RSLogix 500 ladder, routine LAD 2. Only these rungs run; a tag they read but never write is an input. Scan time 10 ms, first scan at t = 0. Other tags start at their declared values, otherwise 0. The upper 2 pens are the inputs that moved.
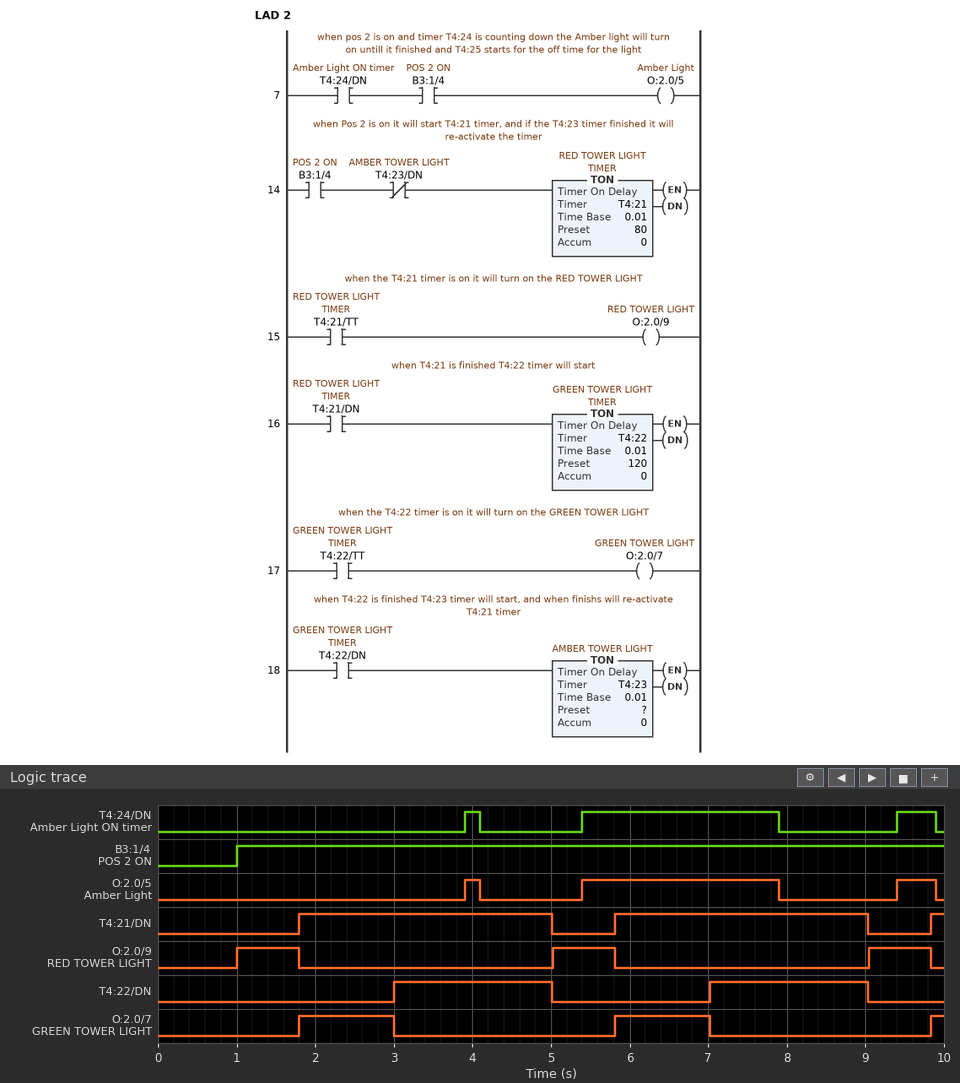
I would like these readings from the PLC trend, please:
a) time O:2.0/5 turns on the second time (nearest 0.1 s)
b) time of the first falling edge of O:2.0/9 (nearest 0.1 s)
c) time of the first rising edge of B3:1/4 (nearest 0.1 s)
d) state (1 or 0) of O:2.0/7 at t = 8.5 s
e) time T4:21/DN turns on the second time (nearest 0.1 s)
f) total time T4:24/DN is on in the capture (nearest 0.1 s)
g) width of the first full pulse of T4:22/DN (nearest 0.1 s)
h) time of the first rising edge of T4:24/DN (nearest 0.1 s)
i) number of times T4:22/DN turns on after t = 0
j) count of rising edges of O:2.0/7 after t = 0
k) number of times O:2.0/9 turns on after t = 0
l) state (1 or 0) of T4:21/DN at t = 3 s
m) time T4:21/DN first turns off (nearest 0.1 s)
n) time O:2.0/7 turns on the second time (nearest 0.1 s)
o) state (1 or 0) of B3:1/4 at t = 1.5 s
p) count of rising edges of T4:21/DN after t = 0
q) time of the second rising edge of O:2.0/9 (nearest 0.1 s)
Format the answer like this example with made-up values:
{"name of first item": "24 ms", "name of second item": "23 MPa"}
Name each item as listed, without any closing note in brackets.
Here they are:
{"time O:2.0/5 turns on the second time": "5.4 s", "time of the first falling edge of O:2.0/9": "1.8 s", "time of the first rising edge of B3:1/4": "1.0 s", "state (1 or 0) of O:2.0/7 at t = 8.5 s": "0", "time T4:21/DN turns on the second time": "5.8 s", "total time T4:24/DN is on in the capture": "3.2 s", "width of the first full pulse of T4:22/DN": "2.0 s", "time of the first rising edge of T4:24/DN": "3.9 s", "number of times T4:22/DN turns on after t = 0": "2", "count of rising edges of O:2.0/7 after t = 0": "3", "number of times O:2.0/9 turns on after t = 0": "3", "state (1 or 0) of T4:21/DN at t = 3 s": "1", "time T4:21/DN first turns off": "5.0 s", "time O:2.0/7 turns on the second time": "5.8 s", "state (1 or 0) of B3:1/4 at t = 1.5 s": "1", "count of rising edges of T4:21/DN after t = 0": "3", "time of the second rising edge of O:2.0/9": "5.0 s"}
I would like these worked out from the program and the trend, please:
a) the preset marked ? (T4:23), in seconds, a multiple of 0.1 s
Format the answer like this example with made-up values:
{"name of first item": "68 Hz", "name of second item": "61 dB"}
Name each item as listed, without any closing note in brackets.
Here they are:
{"the preset marked ? (T4:23), in seconds, a multiple of 0.1 s": "2.0 s"}
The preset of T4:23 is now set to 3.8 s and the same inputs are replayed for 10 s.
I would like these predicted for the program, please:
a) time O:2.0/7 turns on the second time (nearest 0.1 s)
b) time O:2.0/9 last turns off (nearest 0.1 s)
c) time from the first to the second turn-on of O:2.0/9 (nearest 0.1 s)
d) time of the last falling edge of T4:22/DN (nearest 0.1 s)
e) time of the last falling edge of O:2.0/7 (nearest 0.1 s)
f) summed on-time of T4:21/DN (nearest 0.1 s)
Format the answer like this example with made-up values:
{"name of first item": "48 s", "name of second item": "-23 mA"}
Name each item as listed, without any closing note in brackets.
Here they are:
{"time O:2.0/7 turns on the second time": "7.6 s", "time O:2.0/9 last turns off": "7.6 s", "time from the first to the second turn-on of O:2.0/9": "5.8 s", "time of the last falling edge of T4:22/DN": "6.8 s", "time of the last falling edge of O:2.0/7": "8.8 s", "summed on-time of T4:21/DN": "7.4 s"}
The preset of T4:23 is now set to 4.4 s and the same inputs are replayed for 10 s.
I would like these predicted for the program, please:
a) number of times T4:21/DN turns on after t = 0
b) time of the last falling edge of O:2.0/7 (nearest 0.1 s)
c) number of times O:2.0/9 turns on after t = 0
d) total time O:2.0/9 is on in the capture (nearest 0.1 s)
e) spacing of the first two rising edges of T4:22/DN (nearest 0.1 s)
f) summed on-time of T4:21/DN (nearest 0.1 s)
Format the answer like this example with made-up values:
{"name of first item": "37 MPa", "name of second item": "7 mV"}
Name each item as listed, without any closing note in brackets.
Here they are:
{"number of times T4:21/DN turns on after t = 0": "2", "time of the last falling edge of O:2.0/7": "9.4 s", "number of times O:2.0/9 turns on after t = 0": "2", "total time O:2.0/9 is on in the capture": "1.6 s", "spacing of the first two rising edges of T4:22/DN": "6.4 s", "summed on-time of T4:21/DN": "7.4 s"}
